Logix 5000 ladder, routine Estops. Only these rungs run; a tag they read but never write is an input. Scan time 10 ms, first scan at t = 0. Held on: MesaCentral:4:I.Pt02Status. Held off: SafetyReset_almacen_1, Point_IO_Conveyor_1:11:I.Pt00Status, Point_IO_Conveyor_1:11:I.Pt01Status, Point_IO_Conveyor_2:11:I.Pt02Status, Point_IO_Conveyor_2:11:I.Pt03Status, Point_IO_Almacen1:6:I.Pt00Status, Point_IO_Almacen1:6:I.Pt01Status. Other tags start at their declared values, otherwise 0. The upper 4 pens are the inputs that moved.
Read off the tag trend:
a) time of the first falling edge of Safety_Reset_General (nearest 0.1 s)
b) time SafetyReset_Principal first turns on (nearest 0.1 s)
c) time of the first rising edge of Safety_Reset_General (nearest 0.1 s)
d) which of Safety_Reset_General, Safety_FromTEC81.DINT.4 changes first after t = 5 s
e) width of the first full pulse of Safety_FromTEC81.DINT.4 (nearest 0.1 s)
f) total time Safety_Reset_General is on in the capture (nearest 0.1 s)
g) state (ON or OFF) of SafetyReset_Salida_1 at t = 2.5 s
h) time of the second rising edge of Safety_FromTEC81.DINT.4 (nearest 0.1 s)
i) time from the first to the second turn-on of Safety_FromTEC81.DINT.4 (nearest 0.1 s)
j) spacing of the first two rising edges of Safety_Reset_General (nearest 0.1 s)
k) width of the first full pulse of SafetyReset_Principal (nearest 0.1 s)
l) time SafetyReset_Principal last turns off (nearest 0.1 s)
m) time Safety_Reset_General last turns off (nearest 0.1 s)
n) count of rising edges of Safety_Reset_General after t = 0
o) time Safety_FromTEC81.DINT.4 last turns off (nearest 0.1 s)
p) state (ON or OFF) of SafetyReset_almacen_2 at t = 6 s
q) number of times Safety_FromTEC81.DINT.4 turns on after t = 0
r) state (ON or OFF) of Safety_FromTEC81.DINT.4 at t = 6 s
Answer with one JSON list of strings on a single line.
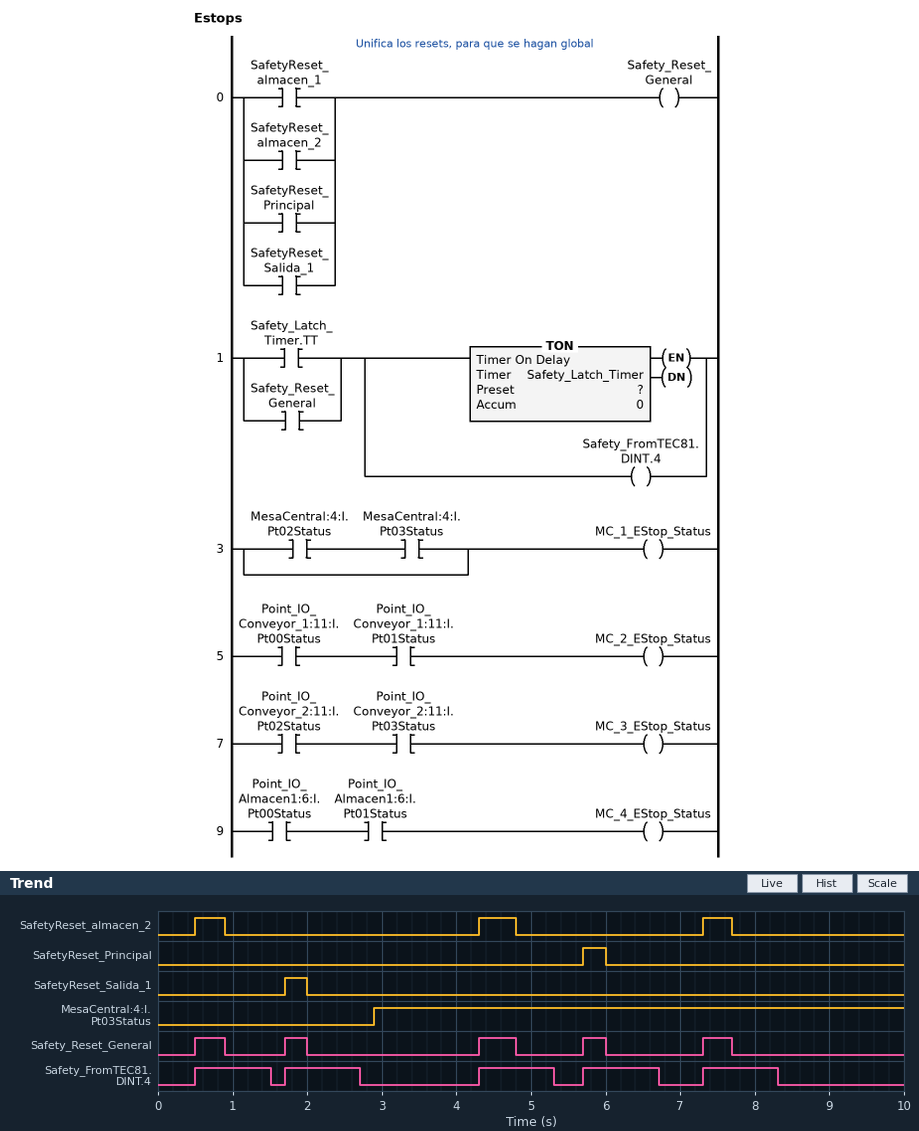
["0.9 s", "5.7 s", "0.5 s", "Safety_FromTEC81.DINT.4", "1.0 s", "1.9 s", "OFF", "1.7 s", "1.2 s", "1.2 s", "0.3 s", "6.0 s", "7.7 s", "5", "8.3 s", "OFF", "5", "ON"]
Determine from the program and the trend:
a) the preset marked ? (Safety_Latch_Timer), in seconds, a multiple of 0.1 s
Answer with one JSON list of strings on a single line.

["1.0 s"]
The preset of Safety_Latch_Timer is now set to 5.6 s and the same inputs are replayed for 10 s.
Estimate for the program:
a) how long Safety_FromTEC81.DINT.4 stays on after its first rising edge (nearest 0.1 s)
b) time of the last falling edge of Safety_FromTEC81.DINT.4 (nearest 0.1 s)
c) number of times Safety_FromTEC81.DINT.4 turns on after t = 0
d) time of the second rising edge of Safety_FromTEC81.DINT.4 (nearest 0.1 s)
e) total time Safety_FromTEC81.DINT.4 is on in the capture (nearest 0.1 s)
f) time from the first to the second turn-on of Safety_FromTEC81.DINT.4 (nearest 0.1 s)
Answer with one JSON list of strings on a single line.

["5.6 s", "6.1 s", "2", "7.3 s", "8.3 s", "6.8 s"]
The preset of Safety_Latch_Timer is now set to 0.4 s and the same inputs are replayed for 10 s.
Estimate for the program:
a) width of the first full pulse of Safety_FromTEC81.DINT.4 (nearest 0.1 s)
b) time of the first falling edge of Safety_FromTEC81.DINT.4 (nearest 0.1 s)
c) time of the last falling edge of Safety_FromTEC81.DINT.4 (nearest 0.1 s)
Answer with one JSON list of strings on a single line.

["0.4 s", "0.9 s", "7.7 s"]
